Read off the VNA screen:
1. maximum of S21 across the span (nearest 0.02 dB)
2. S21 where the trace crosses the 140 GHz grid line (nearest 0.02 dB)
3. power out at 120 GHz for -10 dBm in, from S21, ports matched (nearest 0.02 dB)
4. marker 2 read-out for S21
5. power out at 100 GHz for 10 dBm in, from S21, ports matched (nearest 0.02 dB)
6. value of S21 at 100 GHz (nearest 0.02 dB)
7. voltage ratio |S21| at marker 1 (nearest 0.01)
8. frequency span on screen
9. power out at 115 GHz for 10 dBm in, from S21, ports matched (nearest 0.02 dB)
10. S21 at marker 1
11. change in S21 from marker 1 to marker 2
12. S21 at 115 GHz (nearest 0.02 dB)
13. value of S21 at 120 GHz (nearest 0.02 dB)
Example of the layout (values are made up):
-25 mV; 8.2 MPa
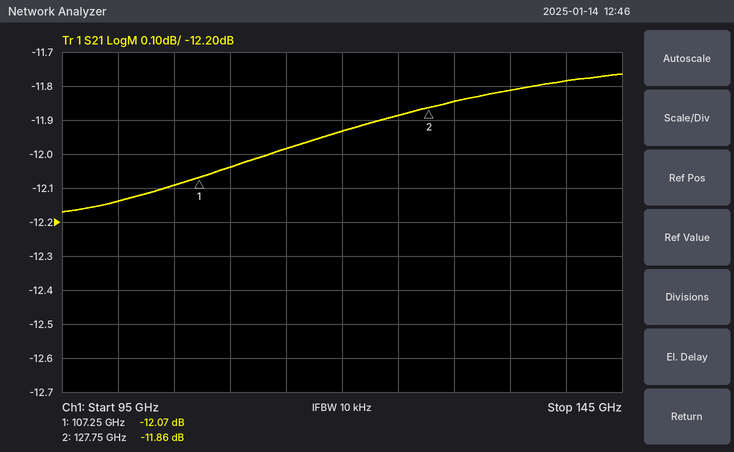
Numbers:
-11.76 dB; -11.78 dB; -21.94 dBm; -11.86 dB; -2.14 dBm; -12.14 dB; 0.25; 50 GHz; -1.98 dBm; -12.07 dB; 0.21 dB; -11.98 dB; -11.94 dB
